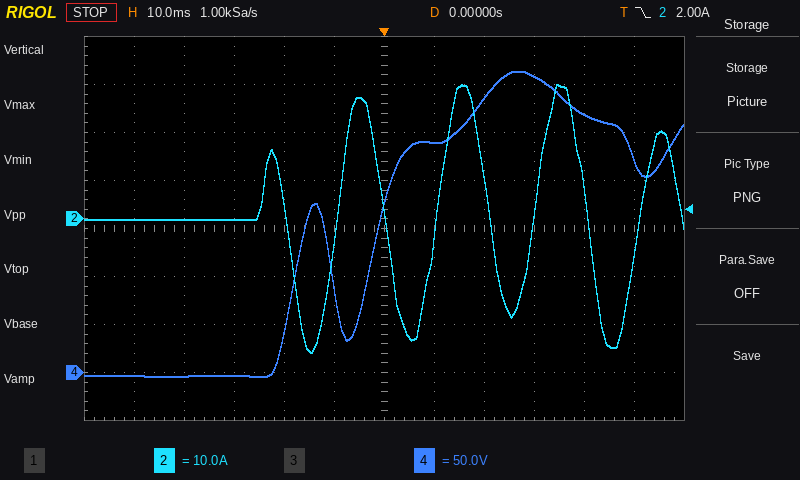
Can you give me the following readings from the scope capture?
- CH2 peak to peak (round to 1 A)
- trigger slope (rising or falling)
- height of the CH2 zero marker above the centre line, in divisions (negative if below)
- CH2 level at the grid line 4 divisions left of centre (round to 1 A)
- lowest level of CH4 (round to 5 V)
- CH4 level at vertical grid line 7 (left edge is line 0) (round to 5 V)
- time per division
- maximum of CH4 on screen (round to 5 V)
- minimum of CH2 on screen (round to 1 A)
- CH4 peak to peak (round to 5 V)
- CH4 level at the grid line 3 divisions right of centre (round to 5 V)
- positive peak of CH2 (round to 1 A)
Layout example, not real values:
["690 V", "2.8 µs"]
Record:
["56 A", "falling", "+0.2 div", "0 A", "-5 V", "240 V", "10 ms", "315 V", "-28 A", "320 V", "310 V", "28 A"]
